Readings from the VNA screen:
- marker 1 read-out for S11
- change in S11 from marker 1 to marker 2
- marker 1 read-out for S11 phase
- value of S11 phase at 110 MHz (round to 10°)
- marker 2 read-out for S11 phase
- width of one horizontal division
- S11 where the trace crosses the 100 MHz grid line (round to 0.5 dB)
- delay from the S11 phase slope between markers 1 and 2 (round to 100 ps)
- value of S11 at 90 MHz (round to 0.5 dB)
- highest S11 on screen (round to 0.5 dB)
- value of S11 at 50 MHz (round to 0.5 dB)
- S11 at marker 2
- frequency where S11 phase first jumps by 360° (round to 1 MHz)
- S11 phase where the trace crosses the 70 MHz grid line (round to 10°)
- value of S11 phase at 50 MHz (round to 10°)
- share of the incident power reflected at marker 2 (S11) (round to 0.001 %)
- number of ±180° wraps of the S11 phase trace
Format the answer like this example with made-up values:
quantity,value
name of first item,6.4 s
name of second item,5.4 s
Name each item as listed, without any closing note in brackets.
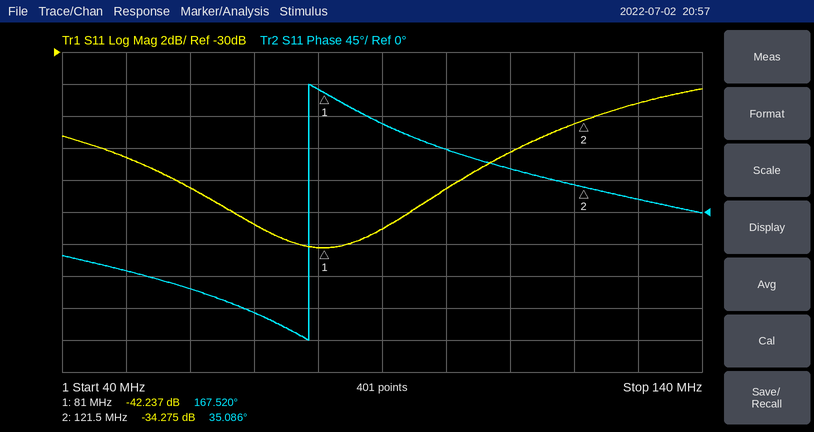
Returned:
quantity,value
marker 1 read-out for S11,-42.237 dB
change in S11 from marker 1 to marker 2,7.962 dB
marker 1 read-out for S11 phase,167.520°
value of S11 phase at 110 MHz,60°
marker 2 read-out for S11 phase,35.086°
width of one horizontal division,10 MHz
S11 where the trace crosses the 100 MHz grid line,-38.5 dB
delay from the S11 phase slope between markers 1 and 2,9.1 ns
value of S11 at 90 MHz,-41.0 dB
highest S11 on screen,-32.5 dB
value of S11 at 50 MHz,-36.5 dB
S11 at marker 2,-34.275 dB
frequency where S11 phase first jumps by 360°,79 MHz
S11 phase where the trace crosses the 70 MHz grid line,-140°
value of S11 phase at 50 MHz,-80°
share of the incident power reflected at marker 2 (S11),0.037 %
number of ±180° wraps of the S11 phase trace,1
